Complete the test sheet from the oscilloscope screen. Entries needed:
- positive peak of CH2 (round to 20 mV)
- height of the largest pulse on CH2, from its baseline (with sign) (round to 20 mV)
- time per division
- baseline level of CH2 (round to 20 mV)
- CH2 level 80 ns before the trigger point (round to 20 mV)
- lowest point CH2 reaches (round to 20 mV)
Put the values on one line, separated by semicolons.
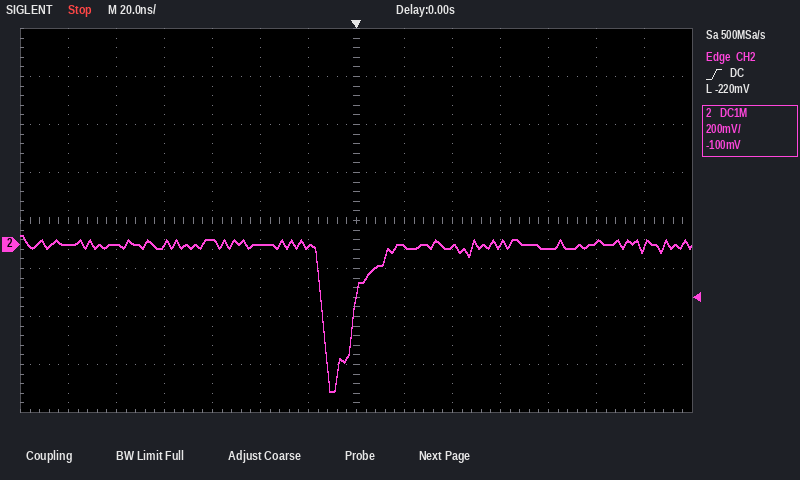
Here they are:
40 mV; -620 mV; 20 ns; 0 mV; 0 mV; -620 mV
